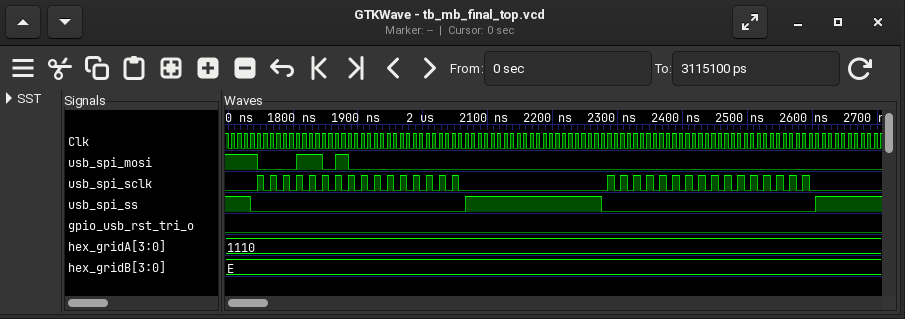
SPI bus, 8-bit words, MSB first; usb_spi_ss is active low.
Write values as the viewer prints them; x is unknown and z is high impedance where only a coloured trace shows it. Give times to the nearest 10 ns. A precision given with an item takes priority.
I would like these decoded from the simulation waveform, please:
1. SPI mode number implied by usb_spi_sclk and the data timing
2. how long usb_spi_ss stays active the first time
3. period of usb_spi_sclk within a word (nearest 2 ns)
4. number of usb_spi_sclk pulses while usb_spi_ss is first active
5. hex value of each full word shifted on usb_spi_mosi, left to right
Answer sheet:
1
330 ns
20 ns
16
1A, 00, 00, 00
